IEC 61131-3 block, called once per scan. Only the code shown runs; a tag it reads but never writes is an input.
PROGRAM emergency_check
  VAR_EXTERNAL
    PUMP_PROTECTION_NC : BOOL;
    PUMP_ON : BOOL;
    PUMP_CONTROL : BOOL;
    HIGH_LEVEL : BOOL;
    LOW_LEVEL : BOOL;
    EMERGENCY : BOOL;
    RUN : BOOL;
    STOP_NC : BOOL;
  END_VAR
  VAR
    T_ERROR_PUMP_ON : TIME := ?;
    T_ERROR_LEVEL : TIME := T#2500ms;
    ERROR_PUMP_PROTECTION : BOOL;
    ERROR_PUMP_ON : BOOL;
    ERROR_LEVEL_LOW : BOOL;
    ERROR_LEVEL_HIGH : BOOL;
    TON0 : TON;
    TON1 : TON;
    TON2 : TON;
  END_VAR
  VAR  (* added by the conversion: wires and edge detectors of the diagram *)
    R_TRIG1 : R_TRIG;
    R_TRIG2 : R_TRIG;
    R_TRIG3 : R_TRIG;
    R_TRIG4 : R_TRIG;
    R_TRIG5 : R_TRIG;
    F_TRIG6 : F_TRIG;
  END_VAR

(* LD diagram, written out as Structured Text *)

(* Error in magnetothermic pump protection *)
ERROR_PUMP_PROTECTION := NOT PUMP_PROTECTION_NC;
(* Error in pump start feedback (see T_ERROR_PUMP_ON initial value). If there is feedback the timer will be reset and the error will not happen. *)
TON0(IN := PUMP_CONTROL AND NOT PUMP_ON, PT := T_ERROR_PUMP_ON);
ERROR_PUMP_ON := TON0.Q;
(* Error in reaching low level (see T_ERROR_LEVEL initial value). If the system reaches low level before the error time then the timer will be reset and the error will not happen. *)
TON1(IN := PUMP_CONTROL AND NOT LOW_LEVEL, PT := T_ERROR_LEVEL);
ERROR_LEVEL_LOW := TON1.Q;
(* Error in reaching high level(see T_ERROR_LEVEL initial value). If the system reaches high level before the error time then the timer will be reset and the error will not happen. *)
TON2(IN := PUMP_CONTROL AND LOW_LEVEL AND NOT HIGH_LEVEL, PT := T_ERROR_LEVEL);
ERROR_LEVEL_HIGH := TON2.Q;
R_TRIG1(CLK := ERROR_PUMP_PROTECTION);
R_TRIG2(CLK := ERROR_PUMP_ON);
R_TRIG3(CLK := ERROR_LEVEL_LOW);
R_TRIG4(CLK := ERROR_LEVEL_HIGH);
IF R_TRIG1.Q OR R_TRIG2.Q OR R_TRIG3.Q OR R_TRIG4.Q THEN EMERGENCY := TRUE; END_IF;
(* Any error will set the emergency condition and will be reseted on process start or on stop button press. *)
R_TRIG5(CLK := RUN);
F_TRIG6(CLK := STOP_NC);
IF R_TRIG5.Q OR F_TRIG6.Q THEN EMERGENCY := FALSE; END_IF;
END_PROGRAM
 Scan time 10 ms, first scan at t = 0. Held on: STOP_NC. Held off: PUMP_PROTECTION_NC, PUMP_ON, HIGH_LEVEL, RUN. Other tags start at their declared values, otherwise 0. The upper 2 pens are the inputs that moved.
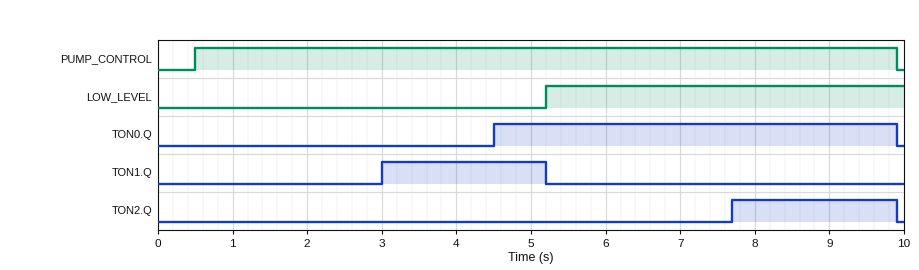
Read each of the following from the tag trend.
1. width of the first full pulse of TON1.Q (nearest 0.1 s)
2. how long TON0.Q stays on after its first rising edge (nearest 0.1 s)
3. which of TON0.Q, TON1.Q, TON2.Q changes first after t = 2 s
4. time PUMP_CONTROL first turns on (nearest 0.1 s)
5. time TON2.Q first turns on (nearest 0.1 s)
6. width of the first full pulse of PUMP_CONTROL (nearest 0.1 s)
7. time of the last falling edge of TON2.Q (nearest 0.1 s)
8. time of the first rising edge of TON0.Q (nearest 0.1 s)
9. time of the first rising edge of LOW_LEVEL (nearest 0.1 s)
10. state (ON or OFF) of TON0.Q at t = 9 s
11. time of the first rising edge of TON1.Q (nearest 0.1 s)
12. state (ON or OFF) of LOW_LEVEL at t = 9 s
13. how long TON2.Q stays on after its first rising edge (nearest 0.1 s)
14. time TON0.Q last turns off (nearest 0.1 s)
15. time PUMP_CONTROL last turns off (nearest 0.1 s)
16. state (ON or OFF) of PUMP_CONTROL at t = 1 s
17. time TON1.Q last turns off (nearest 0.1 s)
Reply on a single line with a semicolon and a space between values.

2.2 s; 5.4 s; TON1.Q; 0.5 s; 7.7 s; 9.4 s; 9.9 s; 4.5 s; 5.2 s; ON; 3.0 s; ON; 2.2 s; 9.9 s; 9.9 s; ON; 5.2 s
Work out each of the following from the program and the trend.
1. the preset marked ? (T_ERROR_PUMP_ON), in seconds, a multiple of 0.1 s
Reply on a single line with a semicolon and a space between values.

4.0 s
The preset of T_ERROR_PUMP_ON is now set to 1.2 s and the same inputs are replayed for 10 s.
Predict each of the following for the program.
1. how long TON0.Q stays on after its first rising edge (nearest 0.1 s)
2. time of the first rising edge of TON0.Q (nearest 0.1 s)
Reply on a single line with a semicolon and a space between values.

8.2 s; 1.7 s
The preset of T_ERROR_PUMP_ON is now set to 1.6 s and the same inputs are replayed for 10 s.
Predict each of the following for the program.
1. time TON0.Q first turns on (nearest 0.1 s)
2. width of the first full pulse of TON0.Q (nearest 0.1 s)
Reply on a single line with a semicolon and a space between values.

2.1 s; 7.8 s
